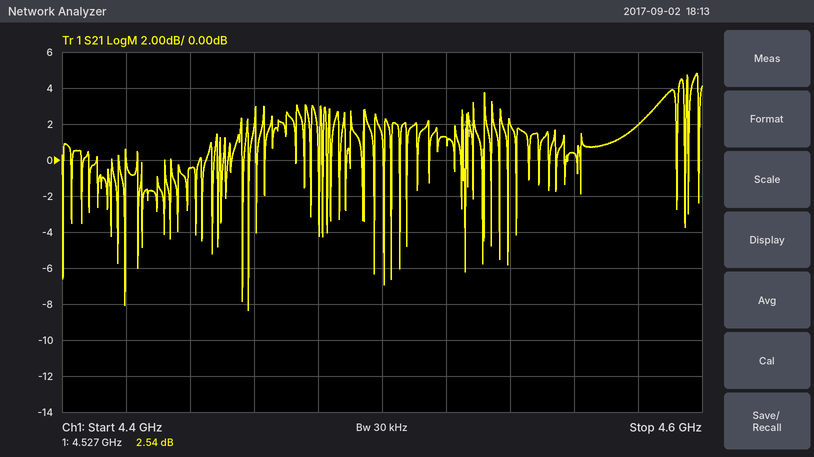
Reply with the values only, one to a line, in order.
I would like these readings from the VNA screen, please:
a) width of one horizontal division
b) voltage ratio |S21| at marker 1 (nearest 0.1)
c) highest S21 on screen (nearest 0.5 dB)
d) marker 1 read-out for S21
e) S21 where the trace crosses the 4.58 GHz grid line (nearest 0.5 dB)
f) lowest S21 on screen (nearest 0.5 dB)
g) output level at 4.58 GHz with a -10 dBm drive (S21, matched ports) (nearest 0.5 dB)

20 MHz
1.3
5.0 dB
2.54 dB
2.0 dB
-8.5 dB
-8.0 dBm
